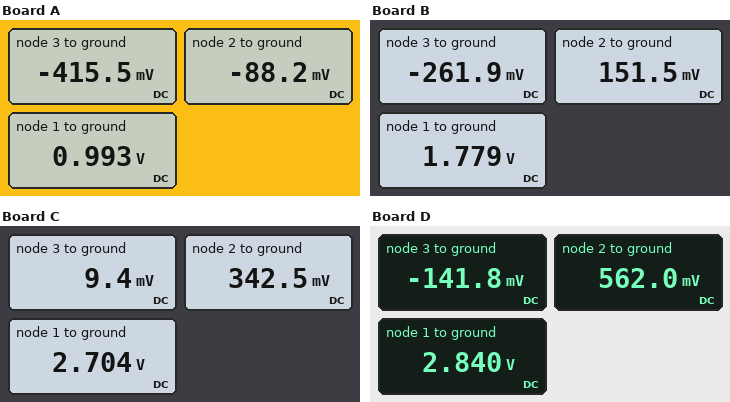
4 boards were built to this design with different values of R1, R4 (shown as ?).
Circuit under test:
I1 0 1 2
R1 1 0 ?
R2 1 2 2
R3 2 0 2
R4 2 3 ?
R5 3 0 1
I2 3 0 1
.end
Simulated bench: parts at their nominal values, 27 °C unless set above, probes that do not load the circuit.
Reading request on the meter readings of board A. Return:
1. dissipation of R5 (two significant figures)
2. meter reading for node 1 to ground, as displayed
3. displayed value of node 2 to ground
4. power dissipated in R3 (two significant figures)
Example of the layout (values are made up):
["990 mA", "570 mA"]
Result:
["170 mW", "0.993 V", "-88.2 mV", "3.9 mW"]
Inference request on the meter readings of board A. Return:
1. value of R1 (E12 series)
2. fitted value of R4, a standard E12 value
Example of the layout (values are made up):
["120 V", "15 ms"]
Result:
["0.68 Ω", "0.56 Ω"]
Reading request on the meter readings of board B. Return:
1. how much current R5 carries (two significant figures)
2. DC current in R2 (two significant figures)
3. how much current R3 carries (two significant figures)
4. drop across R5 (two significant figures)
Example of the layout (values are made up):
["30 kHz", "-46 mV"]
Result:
["260 mA", "810 mA", "76 mA", "260 mV"]
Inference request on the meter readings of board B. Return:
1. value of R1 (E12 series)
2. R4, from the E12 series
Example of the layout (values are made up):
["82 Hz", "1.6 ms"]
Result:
["1.5 Ω", "0.56 Ω"]
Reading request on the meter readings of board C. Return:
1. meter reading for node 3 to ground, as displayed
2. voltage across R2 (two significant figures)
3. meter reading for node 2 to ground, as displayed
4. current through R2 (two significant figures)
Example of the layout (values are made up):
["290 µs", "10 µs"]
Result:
["9.4 mV", "2.4 V", "342.5 mV", "1.2 A"]
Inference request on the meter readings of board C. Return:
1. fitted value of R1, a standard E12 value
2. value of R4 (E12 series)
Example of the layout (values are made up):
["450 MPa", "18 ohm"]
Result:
["3.3 Ω", "0.33 Ω"]
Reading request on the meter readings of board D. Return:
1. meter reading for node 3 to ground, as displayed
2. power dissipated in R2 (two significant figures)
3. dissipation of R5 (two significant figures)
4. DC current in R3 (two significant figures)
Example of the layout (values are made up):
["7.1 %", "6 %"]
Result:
["-141.8 mV", "2.6 W", "20 mW", "280 mA"]
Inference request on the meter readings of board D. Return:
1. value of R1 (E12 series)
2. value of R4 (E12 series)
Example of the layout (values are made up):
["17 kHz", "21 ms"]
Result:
["3.3 Ω", "0.82 Ω"]
